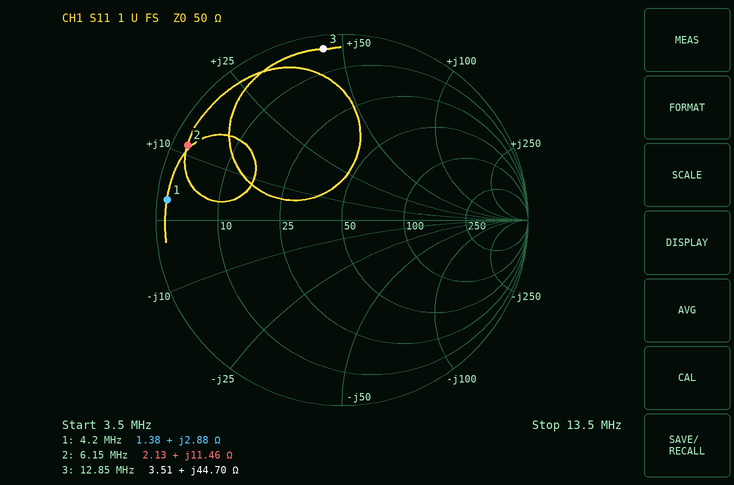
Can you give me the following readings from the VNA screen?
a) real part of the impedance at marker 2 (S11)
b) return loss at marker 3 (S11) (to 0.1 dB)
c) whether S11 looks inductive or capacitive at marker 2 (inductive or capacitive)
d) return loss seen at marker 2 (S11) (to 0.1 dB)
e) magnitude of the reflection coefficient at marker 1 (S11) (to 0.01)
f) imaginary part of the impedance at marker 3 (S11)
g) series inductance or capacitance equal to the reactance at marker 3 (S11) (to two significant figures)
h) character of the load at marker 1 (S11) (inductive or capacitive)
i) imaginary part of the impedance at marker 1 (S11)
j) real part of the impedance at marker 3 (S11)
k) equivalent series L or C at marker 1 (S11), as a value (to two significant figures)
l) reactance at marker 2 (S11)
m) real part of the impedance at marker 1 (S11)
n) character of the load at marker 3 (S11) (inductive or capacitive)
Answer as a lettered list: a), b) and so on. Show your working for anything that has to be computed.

a) 2.13 Ω
b) 0.7 dB
c) inductive
d) 0.7 dB
e) 0.95
f) +44.70 Ω
g) L = 44.7 Ω/(2π × 12.85 MHz) ≈ 554 nH, so 550 nH to two significant figures
h) inductive
i) +2.88 Ω
j) 3.51 Ω
k) L = 2.88 Ω/(2π × 4.2 MHz) ≈ 109 nH, so 110 nH to two significant figures
l) +11.46 Ω
m) 1.38 Ω
n) inductive
